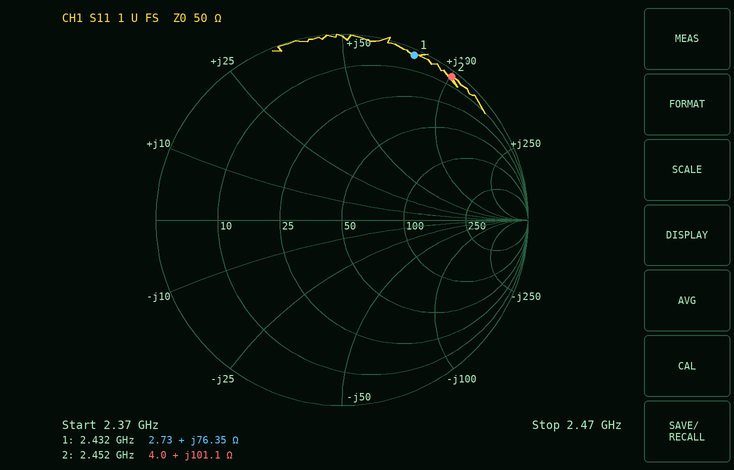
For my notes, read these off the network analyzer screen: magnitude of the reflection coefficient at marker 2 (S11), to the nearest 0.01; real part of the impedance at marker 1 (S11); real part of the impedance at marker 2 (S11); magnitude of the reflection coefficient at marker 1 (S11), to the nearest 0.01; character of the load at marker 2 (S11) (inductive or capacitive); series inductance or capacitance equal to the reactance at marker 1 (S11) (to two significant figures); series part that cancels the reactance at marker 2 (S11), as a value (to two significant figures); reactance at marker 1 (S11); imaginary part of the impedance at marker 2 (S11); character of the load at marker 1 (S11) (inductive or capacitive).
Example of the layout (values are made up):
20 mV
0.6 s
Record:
0.97
2.73 Ω
4.0 Ω
0.97
inductive
5.0 nH
640 fF
+76.35 Ω
+101.1 Ω
inductive
